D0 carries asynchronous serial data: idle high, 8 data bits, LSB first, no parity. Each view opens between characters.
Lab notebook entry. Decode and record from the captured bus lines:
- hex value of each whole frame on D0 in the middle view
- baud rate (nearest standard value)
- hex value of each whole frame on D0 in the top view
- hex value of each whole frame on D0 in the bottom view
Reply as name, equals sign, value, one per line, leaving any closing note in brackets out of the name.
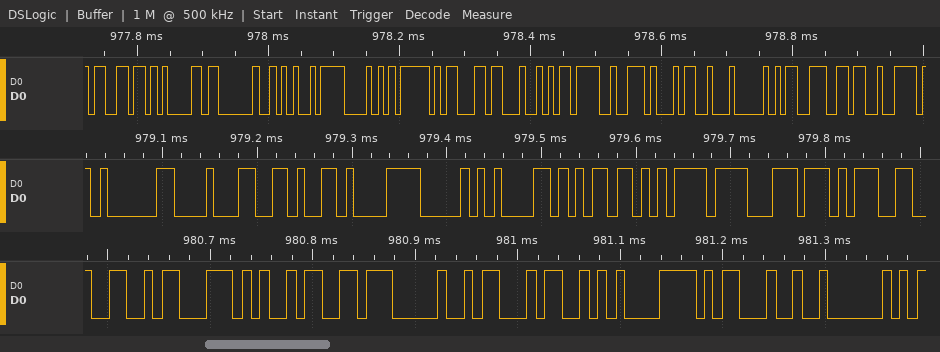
hex value of each whole frame on D0 in the middle view = 81, 88, 96, E1, 50, 58, 5B, EF, DC, 9D
baud rate = 115200 baud
hex value of each whole frame on D0 in the top view = B3, 85, 03, 2A, 0F, F5, 8D, 23, ED, 72, 34, 04, CD, 36
hex value of each whole frame on D0 in the bottom view = A6, 5C, 9A, 07, 1A, 53, 78, 23, 02
